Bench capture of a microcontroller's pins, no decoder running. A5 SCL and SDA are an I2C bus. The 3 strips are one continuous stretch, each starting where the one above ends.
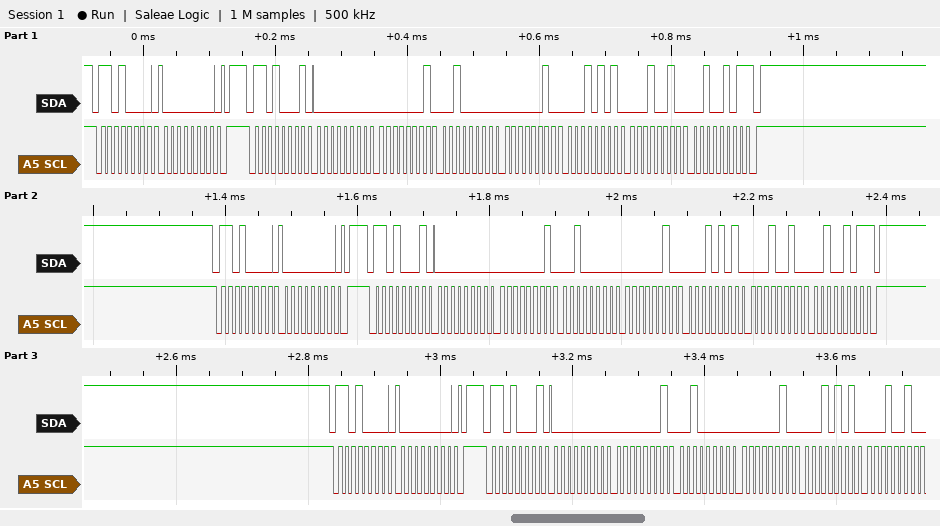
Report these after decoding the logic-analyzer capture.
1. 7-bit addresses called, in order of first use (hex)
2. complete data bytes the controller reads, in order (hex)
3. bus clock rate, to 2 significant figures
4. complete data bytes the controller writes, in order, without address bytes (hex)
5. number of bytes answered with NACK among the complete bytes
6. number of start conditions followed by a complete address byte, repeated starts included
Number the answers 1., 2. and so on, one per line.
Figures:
1. 0x68
2. 00 01 20 02 15 12 25 00 01 20 02 15 12 25 00 01 20 02 15 12
3. 100 kHz
4. 00 00 00
5. 2
6. 6
